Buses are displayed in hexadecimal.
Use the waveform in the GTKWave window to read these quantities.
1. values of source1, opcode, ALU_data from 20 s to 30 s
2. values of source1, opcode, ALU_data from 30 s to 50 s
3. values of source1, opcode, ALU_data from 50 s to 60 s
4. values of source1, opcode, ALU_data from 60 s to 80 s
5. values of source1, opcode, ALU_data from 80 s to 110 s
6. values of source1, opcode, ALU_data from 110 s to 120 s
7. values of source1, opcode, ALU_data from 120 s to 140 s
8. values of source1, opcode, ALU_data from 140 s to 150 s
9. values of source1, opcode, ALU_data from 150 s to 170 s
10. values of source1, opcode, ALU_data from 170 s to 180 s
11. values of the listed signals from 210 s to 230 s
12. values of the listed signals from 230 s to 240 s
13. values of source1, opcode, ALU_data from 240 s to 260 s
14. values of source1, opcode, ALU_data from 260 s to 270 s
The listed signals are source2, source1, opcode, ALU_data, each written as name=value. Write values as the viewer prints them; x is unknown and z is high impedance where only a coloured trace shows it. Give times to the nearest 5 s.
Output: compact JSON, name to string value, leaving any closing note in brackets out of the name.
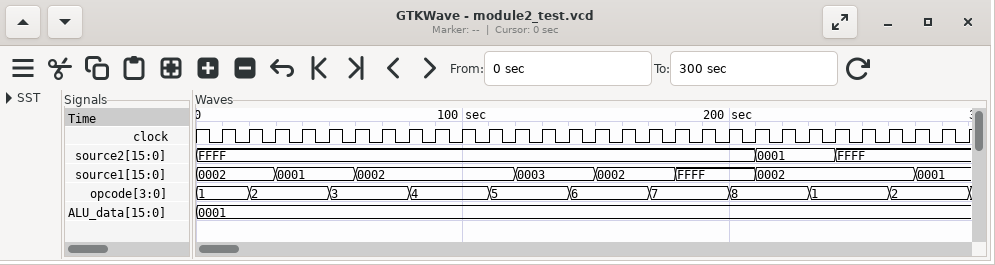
{"values of source1, opcode, ALU_data from 20 s to 30 s": "source1=0002, opcode=2, ALU_data=0001", "values of source1, opcode, ALU_data from 30 s to 50 s": "source1=0001, opcode=2, ALU_data=0001", "values of source1, opcode, ALU_data from 50 s to 60 s": "source1=0001, opcode=3, ALU_data=0001", "values of source1, opcode, ALU_data from 60 s to 80 s": "source1=0002, opcode=3, ALU_data=0001", "values of source1, opcode, ALU_data from 80 s to 110 s": "source1=0002, opcode=4, ALU_data=0001", "values of source1, opcode, ALU_data from 110 s to 120 s": "source1=0002, opcode=5, ALU_data=0001", "values of source1, opcode, ALU_data from 120 s to 140 s": "source1=0003, opcode=5, ALU_data=0001", "values of source1, opcode, ALU_data from 140 s to 150 s": "source1=0003, opcode=6, ALU_data=0001", "values of source1, opcode, ALU_data from 150 s to 170 s": "source1=0002, opcode=6, ALU_data=0001", "values of source1, opcode, ALU_data from 170 s to 180 s": "source1=0002, opcode=7, ALU_data=0001", "values of the listed signals from 210 s to 230 s": "source2=0001, source1=0002, opcode=8, ALU_data=0001", "values of the listed signals from 230 s to 240 s": "source2=0001, source1=0002, opcode=1, ALU_data=0001", "values of source1, opcode, ALU_data from 240 s to 260 s": "source1=0002, opcode=1, ALU_data=0001", "values of source1, opcode, ALU_data from 260 s to 270 s": "source1=0002, opcode=2, ALU_data=0001"}
